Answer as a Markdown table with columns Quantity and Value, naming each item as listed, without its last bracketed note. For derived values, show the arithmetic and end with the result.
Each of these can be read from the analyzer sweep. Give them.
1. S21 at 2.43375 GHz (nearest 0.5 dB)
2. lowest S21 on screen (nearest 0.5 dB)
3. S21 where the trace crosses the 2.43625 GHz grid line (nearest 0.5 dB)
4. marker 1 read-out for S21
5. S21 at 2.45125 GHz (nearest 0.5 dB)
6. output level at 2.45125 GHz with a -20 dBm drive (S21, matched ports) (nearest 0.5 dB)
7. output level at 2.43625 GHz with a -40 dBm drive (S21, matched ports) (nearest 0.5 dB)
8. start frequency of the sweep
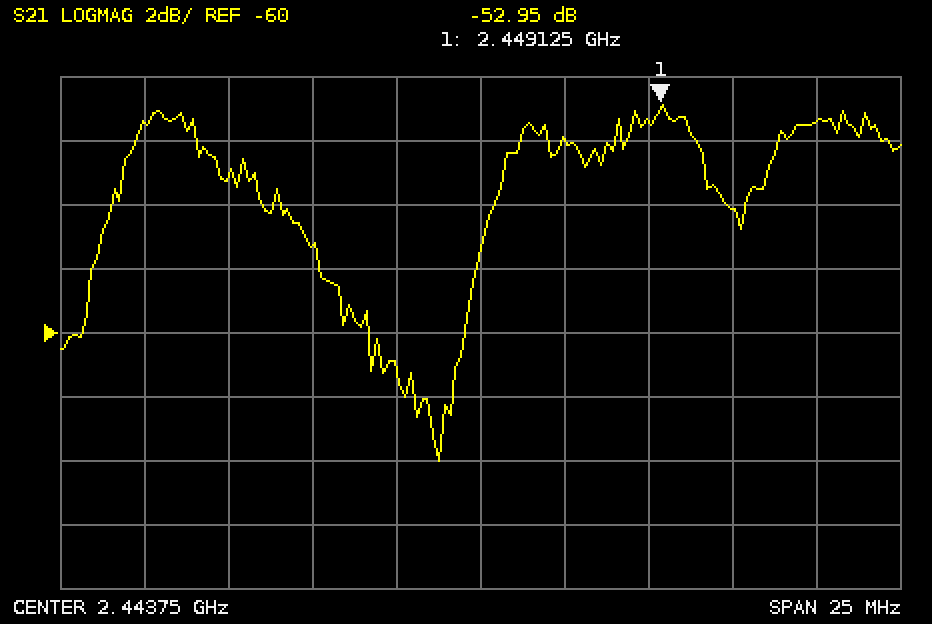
| Quantity | Value |
|---|---|
| S21 at 2.43375 GHz | -53.5 dB |
| lowest S21 on screen | -64.0 dB |
| S21 where the trace crosses the 2.43625 GHz grid line | -55.0 dB |
| marker 1 read-out for S21 | -52.95 dB |
| S21 at 2.45125 GHz | -56.0 dB |
| output level at 2.45125 GHz with a -20 dBm drive (S21, matched ports) | -20 dBm + (-56.0 dB) = -76.0 dBm |
| output level at 2.43625 GHz with a -40 dBm drive (S21, matched ports) | -40 dBm + (-55.0 dB) = -95.0 dBm |
| start frequency of the sweep | 2.43125 GHz |
